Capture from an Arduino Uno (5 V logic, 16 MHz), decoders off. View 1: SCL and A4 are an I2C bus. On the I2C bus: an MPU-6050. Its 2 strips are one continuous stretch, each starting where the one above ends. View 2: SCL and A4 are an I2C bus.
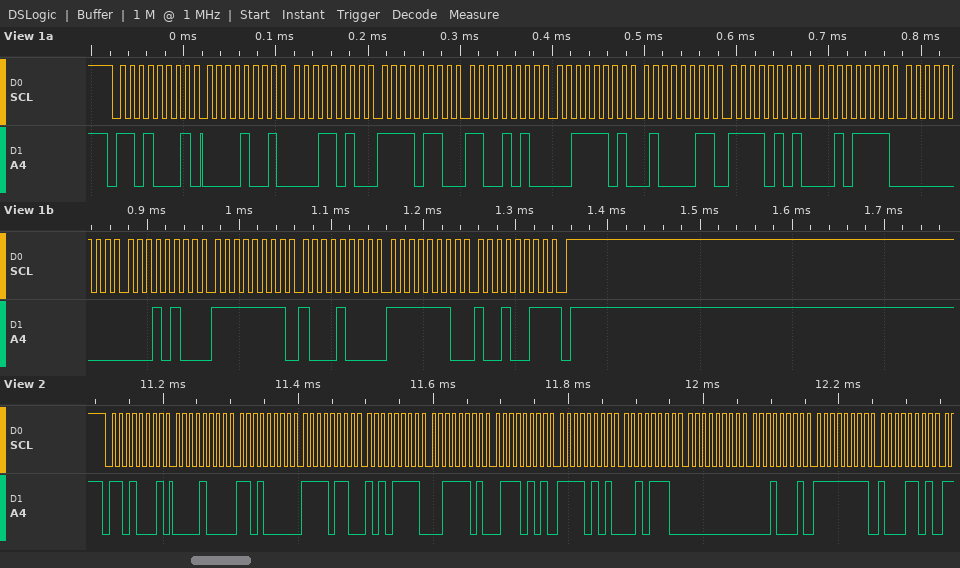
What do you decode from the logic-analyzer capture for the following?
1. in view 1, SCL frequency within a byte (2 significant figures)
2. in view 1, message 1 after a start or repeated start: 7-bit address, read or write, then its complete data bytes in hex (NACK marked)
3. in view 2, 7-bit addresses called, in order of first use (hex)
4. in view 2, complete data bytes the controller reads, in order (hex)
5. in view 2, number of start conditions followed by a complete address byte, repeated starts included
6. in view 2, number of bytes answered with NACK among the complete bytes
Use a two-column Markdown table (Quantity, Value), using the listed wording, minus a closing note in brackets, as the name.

| Quantity | Value |
|---|---|
| in view 1, SCL frequency within a byte | 100 kHz |
| in view 1, message 1 after a start or repeated start: 7-bit address, read or write, then its complete data bytes in hex | 0x68 read: 09 1A F6 CA 3D 43 F5 2F 00 14 FF 88 FE 93 NACK |
| in view 2, 7-bit addresses called, in order of first use | 0x68 |
| in view 2, complete data bytes the controller reads, in order | 08 D0 F6 AF 3D 75 F5 2E 00 11 FF 8D |
| in view 2, number of start conditions followed by a complete address byte, repeated starts included | 1 |
| in view 2, number of bytes answered with NACK among the complete bytes | 0 |
